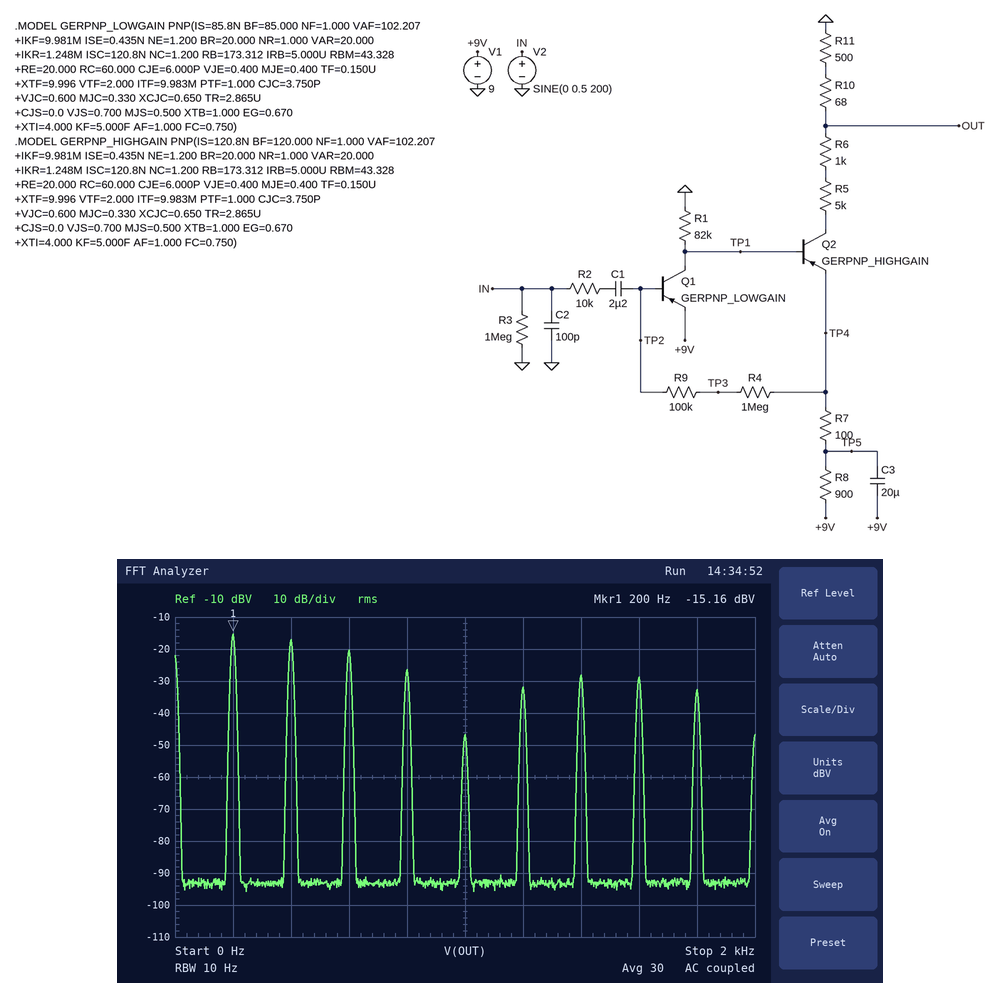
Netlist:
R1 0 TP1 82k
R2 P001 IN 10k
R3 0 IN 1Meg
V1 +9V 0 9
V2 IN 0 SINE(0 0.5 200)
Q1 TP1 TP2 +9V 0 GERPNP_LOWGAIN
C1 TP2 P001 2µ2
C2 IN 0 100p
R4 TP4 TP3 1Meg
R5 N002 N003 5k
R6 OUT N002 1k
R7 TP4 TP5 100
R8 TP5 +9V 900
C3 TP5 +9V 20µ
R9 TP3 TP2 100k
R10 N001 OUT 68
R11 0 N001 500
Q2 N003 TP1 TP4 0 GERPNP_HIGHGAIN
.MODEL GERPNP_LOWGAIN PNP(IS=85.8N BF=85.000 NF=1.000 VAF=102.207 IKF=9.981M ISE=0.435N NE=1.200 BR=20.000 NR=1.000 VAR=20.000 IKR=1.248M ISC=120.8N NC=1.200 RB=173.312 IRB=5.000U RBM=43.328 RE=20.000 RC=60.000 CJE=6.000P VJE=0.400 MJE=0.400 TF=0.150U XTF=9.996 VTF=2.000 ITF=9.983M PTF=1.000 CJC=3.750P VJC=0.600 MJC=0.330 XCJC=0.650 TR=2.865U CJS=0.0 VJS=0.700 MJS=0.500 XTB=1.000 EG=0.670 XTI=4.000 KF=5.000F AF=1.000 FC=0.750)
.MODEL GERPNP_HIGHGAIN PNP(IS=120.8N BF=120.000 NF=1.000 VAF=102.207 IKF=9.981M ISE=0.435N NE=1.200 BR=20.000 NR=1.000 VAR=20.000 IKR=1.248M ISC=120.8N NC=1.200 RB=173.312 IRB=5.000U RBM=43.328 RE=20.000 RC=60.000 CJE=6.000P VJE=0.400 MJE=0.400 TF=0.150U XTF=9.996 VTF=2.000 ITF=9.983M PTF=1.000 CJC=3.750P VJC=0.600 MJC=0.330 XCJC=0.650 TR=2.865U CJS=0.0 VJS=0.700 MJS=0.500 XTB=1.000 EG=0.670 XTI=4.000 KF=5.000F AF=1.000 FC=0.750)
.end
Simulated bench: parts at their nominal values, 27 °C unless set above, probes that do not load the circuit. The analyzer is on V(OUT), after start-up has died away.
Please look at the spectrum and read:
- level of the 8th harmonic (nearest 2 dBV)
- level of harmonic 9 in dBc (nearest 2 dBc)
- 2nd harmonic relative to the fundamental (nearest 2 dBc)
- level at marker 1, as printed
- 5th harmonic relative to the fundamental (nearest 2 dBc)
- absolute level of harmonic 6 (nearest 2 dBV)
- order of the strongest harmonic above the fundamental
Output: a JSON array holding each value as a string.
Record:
["-28 dBV", "-18 dBc", "-2 dBc", "-15.16 dBV", "-32 dBc", "-32 dBV", "2"]
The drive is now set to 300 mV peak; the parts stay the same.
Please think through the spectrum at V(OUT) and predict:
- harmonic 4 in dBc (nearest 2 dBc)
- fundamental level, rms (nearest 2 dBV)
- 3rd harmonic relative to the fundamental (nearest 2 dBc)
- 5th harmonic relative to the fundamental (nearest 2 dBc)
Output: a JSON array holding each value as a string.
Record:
["-16 dBc", "-14 dBV", "-6 dBc", "-22 dBc"]
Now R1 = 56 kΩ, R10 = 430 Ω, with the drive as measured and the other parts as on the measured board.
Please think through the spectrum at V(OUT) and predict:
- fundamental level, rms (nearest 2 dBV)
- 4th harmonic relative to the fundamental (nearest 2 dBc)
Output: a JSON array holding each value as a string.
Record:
["-12 dBV", "-10 dBc"]
